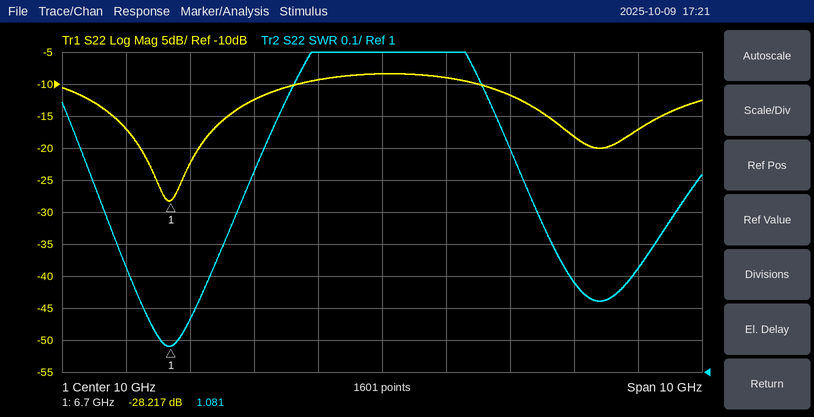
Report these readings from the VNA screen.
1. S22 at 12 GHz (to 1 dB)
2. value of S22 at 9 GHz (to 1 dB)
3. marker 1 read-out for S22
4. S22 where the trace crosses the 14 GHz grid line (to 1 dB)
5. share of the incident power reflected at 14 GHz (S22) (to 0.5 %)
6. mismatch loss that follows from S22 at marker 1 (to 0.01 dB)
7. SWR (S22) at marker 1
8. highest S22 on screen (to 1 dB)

-12 dB
-9 dB
-28.217 dB
-17 dB
2.0 %
0.01 dB
1.081
-8 dB
